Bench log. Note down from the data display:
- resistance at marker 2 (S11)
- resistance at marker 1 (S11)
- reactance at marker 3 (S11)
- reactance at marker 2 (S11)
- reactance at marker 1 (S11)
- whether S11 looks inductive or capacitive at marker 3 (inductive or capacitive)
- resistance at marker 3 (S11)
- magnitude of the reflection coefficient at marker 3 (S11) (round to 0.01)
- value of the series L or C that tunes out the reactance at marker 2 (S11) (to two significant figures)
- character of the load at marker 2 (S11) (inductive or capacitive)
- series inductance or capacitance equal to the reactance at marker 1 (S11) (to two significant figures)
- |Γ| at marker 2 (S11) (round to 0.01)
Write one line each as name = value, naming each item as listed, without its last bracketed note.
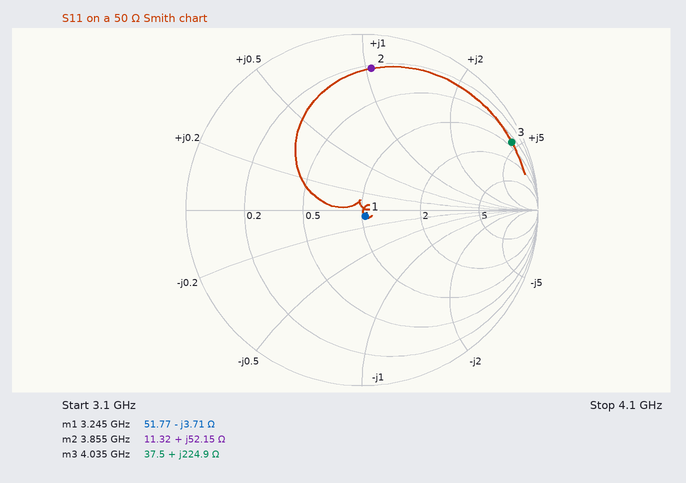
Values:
resistance at marker 2 = 11.32 Ω
resistance at marker 1 = 51.77 Ω
reactance at marker 3 = +224.9 Ω
reactance at marker 2 = +52.15 Ω
reactance at marker 1 = -3.71 Ω
whether S11 looks inductive or capacitive at marker 3 = inductive
resistance at marker 3 = 37.5 Ω
magnitude of the reflection coefficient at marker 3 (S11) = 0.93
value of the series L or C that tunes out the reactance at marker 2 (S11) = 790 fF
character of the load at marker 2 (S11) = inductive
series inductance or capacitance equal to the reactance at marker 1 (S11) = 13 pF
|Γ| at marker 2 (S11) = 0.81
